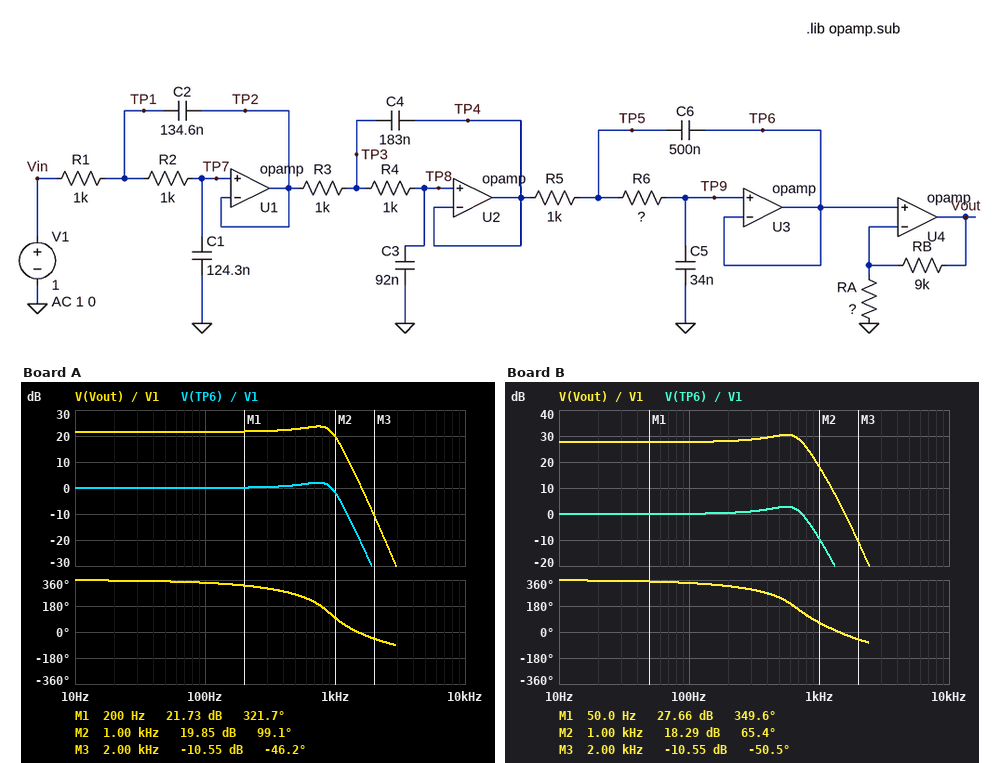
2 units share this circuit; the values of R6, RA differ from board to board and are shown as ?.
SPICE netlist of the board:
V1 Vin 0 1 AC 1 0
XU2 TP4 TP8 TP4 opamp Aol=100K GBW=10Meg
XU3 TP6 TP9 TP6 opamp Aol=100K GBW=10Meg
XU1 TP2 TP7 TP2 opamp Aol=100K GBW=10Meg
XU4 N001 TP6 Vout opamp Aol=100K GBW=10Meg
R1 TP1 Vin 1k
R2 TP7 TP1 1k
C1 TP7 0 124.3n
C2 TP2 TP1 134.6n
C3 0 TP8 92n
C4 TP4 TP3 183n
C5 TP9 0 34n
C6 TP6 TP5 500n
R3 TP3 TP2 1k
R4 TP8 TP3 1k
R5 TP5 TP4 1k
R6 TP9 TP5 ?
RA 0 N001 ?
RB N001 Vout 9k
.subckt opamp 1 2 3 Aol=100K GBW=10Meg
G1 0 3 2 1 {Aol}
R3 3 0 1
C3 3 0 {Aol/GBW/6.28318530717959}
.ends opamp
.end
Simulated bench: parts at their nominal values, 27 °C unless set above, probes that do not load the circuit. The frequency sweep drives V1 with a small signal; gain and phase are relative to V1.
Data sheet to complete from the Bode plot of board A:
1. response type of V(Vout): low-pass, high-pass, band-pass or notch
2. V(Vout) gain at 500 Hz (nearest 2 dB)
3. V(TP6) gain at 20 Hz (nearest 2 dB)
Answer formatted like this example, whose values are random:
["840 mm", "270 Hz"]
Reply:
["low-pass", "22 dB", "0 dB"]
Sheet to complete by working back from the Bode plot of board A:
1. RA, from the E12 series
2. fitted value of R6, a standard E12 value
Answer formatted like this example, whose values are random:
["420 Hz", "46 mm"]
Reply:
["820 Ω", "1.8 kΩ"]
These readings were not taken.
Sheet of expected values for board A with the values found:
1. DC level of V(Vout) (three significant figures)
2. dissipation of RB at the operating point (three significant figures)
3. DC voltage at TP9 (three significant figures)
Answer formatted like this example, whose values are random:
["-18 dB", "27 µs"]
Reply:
["12.0 V", "13.4 mW", "1.00 V"]
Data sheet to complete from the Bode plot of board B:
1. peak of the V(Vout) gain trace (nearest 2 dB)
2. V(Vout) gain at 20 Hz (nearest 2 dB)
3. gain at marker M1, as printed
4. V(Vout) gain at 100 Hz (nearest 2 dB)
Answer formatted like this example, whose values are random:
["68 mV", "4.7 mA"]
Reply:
["30 dB", "28 dB", "27.66 dB", "28 dB"]
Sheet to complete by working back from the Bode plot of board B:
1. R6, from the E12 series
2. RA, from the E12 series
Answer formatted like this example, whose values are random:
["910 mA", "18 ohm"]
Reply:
["3.3 kΩ", "390 Ω"]
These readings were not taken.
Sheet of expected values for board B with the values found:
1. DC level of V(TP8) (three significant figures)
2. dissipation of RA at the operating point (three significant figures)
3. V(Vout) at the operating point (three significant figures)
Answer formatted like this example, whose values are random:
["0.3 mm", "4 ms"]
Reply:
["1.00 V", "2.56 mW", "24.1 V"]
